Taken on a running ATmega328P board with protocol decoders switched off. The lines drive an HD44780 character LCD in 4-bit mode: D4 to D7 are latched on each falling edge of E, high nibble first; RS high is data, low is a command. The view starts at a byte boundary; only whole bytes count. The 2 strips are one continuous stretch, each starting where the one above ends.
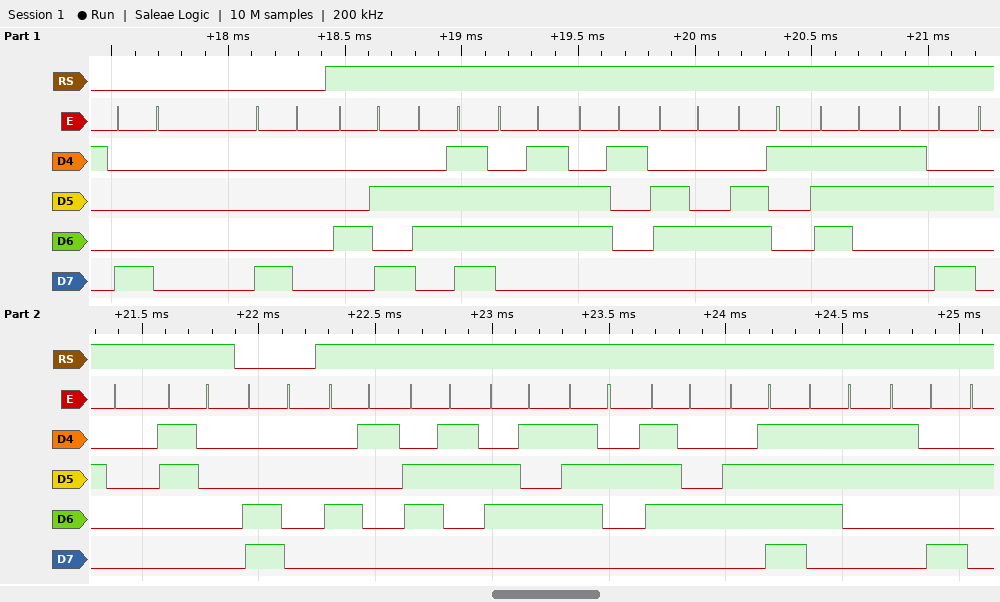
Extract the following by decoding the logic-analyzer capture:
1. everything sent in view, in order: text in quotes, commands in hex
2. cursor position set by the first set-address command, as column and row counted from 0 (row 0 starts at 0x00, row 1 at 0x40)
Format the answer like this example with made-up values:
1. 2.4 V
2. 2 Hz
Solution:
1. 0x80 0x80 "Jogadas: 0" 0xC0 "Acertos:"
2. column 0, row 0
